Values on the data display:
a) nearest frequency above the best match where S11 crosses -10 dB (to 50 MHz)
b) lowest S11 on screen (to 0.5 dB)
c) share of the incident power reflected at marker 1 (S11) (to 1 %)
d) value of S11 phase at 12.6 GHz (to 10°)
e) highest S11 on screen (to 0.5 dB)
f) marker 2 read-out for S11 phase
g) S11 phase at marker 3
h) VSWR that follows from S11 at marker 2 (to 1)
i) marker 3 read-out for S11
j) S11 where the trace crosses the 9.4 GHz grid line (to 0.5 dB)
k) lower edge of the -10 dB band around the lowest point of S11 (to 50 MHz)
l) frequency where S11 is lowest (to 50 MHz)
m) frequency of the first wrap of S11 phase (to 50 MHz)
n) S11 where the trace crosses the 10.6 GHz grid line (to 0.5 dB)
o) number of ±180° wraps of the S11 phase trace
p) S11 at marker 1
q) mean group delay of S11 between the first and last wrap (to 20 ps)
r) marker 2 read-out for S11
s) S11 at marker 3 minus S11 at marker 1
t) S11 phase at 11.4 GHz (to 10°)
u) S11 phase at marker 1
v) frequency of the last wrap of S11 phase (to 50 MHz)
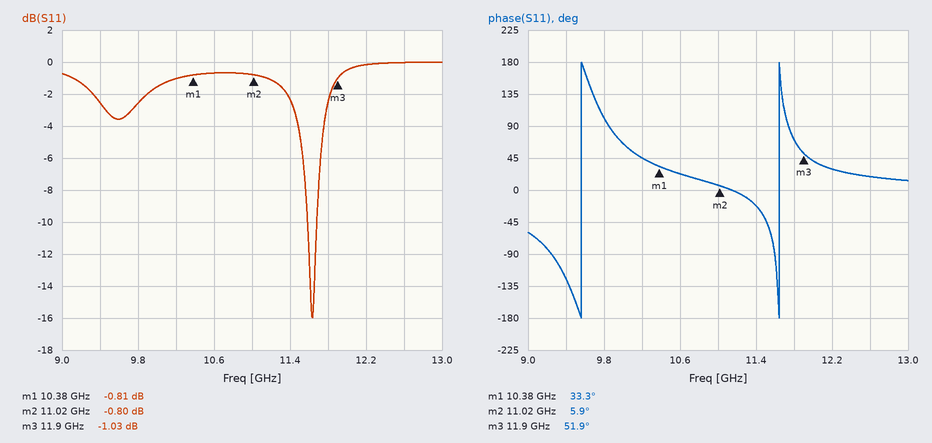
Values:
11.70 GHz
-16.0 dB
83 %
20°
0.0 dB
5.9°
51.9°
22
-1.03 dB
-2.5 dB
11.60 GHz
11.65 GHz
9.55 GHz
-0.5 dB
2
-0.81 dB
480 ps
-0.80 dB
-0.22 dB
-20°
33.3°
11.65 GHz
